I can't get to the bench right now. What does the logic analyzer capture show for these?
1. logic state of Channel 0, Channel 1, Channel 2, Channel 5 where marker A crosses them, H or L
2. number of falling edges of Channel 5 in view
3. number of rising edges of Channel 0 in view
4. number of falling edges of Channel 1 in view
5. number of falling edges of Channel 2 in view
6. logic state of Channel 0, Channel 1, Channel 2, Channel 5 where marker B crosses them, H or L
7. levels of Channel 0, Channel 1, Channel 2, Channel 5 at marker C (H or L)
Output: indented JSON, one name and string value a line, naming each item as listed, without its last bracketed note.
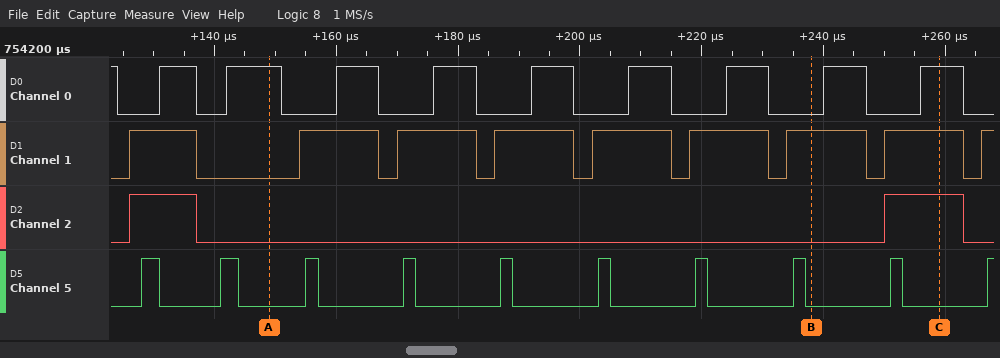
{
  "logic state of Channel 0, Channel 1, Channel 2, Channel 5 where marker A crosses them, H or L": "Channel 0=H, Channel 1=L, Channel 2=L, Channel 5=L",
  "number of falling edges of Channel 5 in view": "9",
  "number of rising edges of Channel 0 in view": "9",
  "number of falling edges of Channel 1 in view": "8",
  "number of falling edges of Channel 2 in view": "2",
  "logic state of Channel 0, Channel 1, Channel 2, Channel 5 where marker B crosses them, H or L": "Channel 0=L, Channel 1=H, Channel 2=L, Channel 5=L",
  "levels of Channel 0, Channel 1, Channel 2, Channel 5 at marker C": "Channel 0=H, Channel 1=H, Channel 2=H, Channel 5=L"
}
